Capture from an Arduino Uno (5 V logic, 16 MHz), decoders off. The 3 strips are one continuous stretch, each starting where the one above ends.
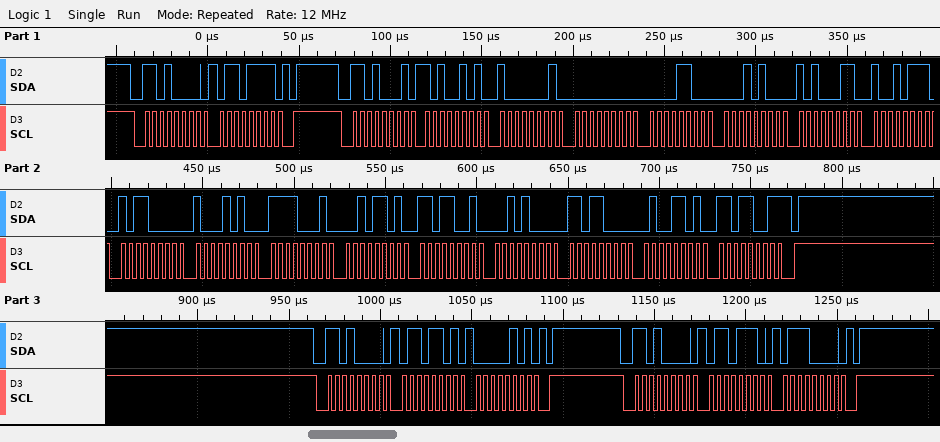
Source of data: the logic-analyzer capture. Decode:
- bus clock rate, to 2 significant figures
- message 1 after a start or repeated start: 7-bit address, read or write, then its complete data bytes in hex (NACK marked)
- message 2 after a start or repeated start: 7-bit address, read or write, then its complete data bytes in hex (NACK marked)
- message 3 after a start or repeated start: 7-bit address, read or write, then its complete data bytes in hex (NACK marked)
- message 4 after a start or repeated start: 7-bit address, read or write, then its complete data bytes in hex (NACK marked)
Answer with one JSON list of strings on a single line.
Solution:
["250 kHz", "0x68 write: 6F", "0x68 read: A5 81 00 0C 14 A3 97 B0 8A F1 2D D9 28 D8 4D D9 NACK", "0x68 write: 6D 05", "0x68 write: 6E 70"]
